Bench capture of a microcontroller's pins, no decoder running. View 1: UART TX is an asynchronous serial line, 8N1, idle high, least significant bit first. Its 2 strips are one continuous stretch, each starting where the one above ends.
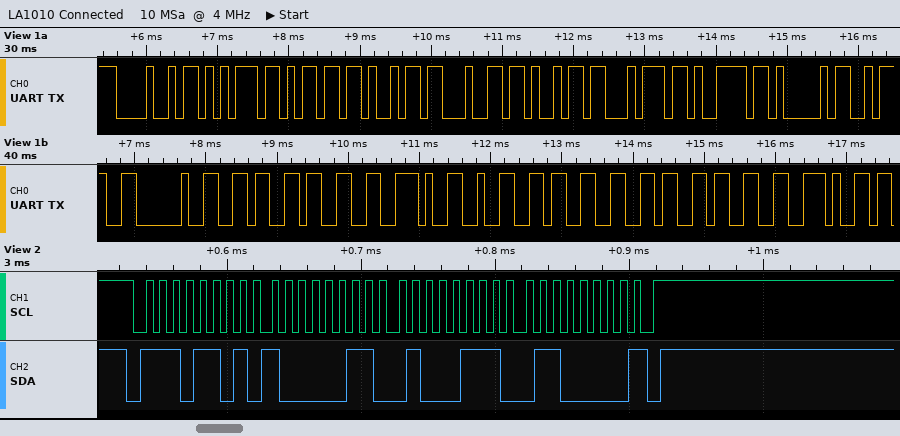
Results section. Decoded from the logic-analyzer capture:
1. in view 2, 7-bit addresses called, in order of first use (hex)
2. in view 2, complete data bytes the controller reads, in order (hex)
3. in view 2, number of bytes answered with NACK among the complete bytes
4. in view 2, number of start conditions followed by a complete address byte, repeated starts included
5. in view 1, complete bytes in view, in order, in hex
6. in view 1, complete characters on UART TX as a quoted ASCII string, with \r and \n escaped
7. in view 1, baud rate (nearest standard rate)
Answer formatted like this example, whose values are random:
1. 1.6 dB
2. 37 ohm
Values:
1. 0x76
2. 83 47 60
3. 1
4. 1
5. 0x48 0x75 0x6D 0x69 0x64 0x69 0x74 0x79 0x41 0x3A 0x20 0x36 0x33 0x2E 0x32 0x33 0x36 0x33 0x2E
6. "HumidityA: 63.2363."
7. 9600 baud
